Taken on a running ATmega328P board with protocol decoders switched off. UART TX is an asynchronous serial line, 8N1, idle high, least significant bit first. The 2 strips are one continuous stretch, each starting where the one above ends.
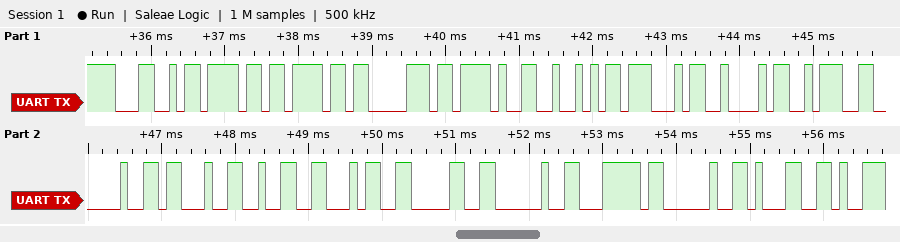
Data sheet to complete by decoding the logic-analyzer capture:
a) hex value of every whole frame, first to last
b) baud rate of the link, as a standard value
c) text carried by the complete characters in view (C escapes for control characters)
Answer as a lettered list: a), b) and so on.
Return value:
a) 4C 6F 6F 70 2F 52 47 42 3A 20 23 32 34 30 20 7C 20 31
b) 9600 baud
c) "Loop/RGB: #240 | 1"
